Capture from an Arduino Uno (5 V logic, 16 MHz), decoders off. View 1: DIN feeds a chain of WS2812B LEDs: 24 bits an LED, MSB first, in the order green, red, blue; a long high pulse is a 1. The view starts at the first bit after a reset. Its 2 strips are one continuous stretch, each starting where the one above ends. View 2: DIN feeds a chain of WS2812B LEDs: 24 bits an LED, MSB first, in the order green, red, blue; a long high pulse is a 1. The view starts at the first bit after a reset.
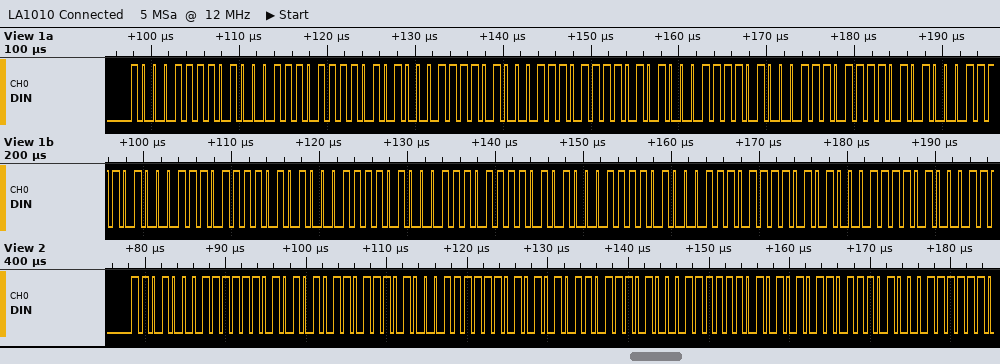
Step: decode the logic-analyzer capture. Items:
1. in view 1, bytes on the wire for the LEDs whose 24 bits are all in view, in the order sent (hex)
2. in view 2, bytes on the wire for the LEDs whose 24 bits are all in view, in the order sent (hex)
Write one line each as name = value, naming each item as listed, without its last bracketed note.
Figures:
in view 1, bytes on the wire for the LEDs whose 24 bits are all in view, in the order sent = 8F 47 7A 8F 47 7A 8F 47 7A 8F 47 7A 8F 47 7A 8F 47 7A
in view 2, bytes on the wire for the LEDs whose 24 bits are all in view, in the order sent = D1 FA AD D1 FA AD D1 FA AD
